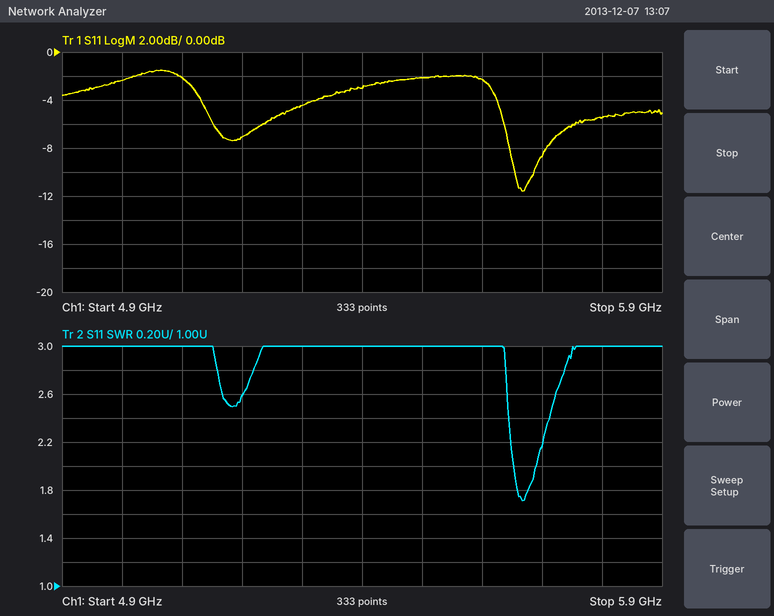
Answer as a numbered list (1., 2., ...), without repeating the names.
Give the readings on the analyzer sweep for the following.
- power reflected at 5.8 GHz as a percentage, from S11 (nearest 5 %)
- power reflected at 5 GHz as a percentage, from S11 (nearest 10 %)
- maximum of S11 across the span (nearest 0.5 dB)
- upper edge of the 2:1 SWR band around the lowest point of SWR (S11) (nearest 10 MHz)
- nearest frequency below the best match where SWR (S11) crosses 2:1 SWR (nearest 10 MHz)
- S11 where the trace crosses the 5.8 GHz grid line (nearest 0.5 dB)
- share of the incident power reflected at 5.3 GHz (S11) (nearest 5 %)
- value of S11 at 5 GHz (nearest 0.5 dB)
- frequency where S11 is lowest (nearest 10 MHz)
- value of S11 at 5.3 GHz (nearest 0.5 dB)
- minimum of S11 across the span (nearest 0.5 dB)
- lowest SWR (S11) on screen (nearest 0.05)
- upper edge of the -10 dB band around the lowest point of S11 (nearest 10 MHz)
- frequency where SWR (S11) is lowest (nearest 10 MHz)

1. 30 %
2. 60 %
3. -1.5 dB
4. 5.69 GHz
5. 5.65 GHz
6. -5.5 dB
7. 35 %
8. -2.5 dB
9. 5.67 GHz
10. -4.5 dB
11. -11.5 dB
12. 1.70
13. 5.69 GHz
14. 5.67 GHz
